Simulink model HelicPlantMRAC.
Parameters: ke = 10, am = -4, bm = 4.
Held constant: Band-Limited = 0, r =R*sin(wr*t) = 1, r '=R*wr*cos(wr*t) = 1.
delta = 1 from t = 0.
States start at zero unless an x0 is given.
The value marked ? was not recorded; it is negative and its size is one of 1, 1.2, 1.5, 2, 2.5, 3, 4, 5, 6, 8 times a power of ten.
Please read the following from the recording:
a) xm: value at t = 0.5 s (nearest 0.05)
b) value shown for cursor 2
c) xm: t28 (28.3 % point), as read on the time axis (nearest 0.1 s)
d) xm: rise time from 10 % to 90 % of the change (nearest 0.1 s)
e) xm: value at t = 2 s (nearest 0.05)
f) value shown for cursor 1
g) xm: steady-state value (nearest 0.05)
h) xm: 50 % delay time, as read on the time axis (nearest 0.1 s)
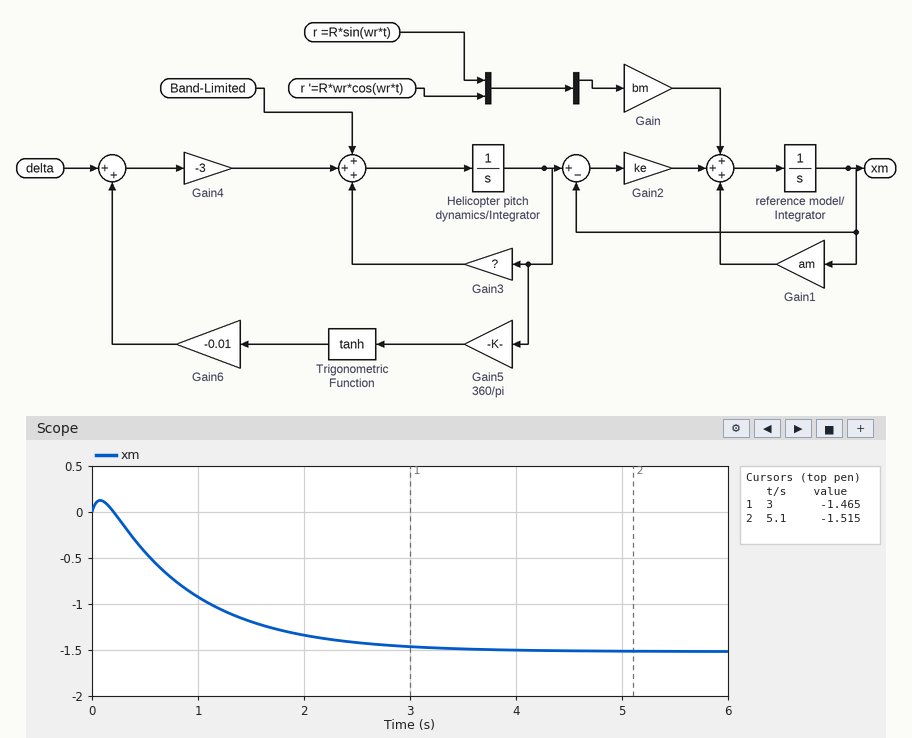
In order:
-0.45
-1.515
0.5 s
1.8 s
-1.35
-1.465
-1.50
0.8 s
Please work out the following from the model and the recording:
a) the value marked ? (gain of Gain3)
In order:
-1.2
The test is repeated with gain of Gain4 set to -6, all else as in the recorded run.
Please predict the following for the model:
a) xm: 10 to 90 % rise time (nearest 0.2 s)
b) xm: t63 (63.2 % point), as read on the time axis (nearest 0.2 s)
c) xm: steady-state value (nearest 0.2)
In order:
1.8 s
1.0 s
-3.4
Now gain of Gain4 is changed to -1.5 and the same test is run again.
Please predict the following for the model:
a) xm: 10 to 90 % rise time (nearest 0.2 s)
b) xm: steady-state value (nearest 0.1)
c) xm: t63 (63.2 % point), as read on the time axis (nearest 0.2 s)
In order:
1.8 s
-0.6
1.2 s
